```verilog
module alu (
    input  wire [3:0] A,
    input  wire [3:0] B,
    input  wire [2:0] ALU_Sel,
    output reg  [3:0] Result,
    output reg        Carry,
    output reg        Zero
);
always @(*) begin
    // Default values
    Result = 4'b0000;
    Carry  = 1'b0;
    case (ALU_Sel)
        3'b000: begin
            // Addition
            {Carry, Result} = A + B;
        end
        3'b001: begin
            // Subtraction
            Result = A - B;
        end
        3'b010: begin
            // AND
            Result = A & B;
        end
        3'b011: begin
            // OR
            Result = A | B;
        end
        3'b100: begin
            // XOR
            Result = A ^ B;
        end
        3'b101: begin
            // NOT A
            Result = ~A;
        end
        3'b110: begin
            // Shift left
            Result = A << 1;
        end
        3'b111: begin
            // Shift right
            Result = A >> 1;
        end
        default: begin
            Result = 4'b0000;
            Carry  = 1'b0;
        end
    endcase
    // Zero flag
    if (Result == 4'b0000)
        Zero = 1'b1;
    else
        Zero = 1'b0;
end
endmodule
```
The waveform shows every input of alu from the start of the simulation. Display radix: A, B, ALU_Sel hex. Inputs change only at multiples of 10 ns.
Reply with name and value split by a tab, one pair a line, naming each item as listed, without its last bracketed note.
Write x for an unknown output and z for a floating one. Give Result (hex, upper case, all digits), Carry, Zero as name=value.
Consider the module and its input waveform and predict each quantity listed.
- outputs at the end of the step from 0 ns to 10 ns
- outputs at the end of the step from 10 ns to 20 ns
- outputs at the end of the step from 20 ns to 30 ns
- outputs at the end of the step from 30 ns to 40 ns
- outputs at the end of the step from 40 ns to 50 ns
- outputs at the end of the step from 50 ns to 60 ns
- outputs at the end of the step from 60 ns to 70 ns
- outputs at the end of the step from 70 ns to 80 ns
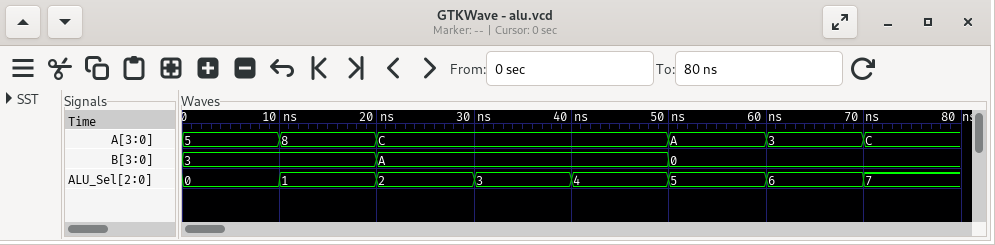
outputs at the end of the step from 0 ns to 10 ns	Result=8, Carry=0, Zero=0
outputs at the end of the step from 10 ns to 20 ns	Result=5, Carry=0, Zero=0
outputs at the end of the step from 20 ns to 30 ns	Result=8, Carry=0, Zero=0
outputs at the end of the step from 30 ns to 40 ns	Result=E, Carry=0, Zero=0
outputs at the end of the step from 40 ns to 50 ns	Result=6, Carry=0, Zero=0
outputs at the end of the step from 50 ns to 60 ns	Result=5, Carry=0, Zero=0
outputs at the end of the step from 60 ns to 70 ns	Result=6, Carry=0, Zero=0
outputs at the end of the step from 70 ns to 80 ns	Result=6, Carry=0, Zero=0
